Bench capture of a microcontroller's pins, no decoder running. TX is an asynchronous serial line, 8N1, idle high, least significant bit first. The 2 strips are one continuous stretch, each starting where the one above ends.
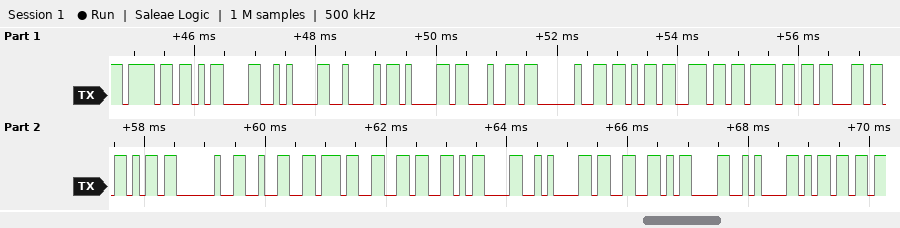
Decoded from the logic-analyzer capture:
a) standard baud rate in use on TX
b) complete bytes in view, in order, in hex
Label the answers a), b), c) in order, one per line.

a) 9600 baud
b) 0x6F 0x0D 0x0A 0x42 0x61 0x64 0x20 0x6B 0x6E 0x6F 0x63 0x6B 0x20 0x32 0x37 0x36 0x0D 0x0A 0x33 0x0D 0x0A 0x6D
